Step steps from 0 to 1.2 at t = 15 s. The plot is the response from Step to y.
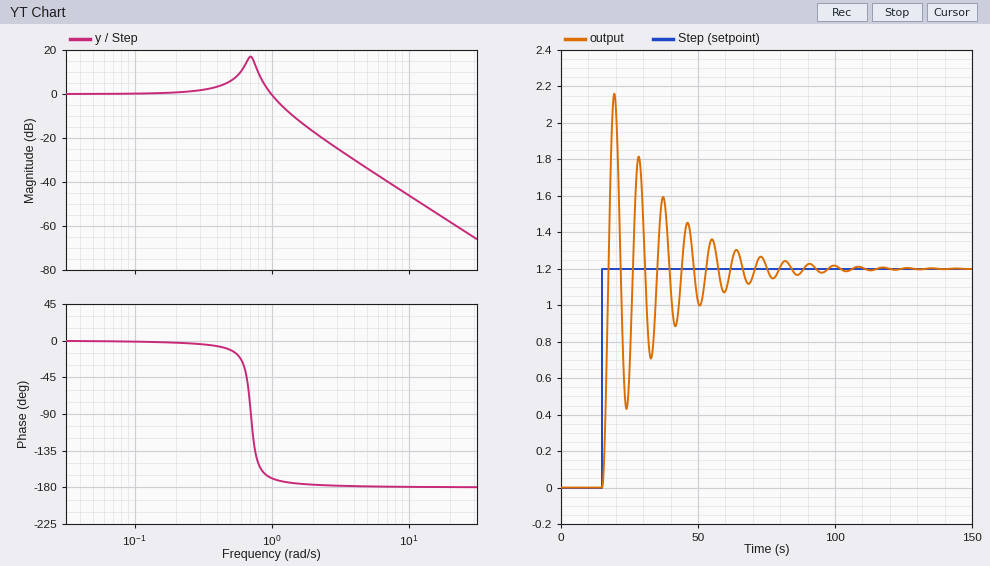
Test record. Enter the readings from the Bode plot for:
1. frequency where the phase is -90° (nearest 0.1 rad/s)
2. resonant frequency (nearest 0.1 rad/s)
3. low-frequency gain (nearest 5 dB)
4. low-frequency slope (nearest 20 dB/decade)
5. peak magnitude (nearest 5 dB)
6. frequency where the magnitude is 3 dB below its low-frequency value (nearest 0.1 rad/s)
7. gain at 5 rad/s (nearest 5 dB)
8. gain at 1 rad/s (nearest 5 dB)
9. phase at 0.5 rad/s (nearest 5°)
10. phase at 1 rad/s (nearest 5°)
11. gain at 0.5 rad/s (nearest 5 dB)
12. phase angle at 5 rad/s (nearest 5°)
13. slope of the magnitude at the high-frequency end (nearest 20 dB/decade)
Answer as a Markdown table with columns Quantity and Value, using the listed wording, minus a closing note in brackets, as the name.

| Quantity | Value |
|---|---|
| frequency where the phase is -90° | 0.7 rad/s |
| resonant frequency | 0.7 rad/s |
| low-frequency gain | 0 dB |
| low-frequency slope | 0 dB/decade |
| peak magnitude | 15 dB |
| frequency where the magnitude is 3 dB below its low-frequency value | 1.1 rad/s |
| gain at 5 rad/s | -35 dB |
| gain at 1 rad/s | 0 dB |
| phase at 0.5 rad/s | -10° |
| phase at 1 rad/s | -170° |
| gain at 0.5 rad/s | 5 dB |
| phase angle at 5 rad/s | -180° |
| slope of the magnitude at the high-frequency end | -40 dB/decade |
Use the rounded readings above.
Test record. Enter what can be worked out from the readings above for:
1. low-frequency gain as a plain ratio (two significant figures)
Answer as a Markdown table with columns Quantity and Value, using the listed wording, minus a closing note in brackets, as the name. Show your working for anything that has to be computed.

| Quantity | Value |
|---|---|
| low-frequency gain as a plain ratio | 10^(0 / 20) = 1.0 |
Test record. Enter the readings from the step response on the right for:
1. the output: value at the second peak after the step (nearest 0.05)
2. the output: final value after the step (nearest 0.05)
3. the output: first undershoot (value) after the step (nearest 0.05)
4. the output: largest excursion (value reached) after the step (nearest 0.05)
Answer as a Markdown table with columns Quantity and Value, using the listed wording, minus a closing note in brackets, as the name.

| Quantity | Value |
|---|---|
| the output: value at the second peak after the step | 1.80 |
| the output: final value after the step | 1.20 |
| the output: first undershoot (value) after the step | 0.45 |
| the output: largest excursion (value reached) after the step | 2.15 |
